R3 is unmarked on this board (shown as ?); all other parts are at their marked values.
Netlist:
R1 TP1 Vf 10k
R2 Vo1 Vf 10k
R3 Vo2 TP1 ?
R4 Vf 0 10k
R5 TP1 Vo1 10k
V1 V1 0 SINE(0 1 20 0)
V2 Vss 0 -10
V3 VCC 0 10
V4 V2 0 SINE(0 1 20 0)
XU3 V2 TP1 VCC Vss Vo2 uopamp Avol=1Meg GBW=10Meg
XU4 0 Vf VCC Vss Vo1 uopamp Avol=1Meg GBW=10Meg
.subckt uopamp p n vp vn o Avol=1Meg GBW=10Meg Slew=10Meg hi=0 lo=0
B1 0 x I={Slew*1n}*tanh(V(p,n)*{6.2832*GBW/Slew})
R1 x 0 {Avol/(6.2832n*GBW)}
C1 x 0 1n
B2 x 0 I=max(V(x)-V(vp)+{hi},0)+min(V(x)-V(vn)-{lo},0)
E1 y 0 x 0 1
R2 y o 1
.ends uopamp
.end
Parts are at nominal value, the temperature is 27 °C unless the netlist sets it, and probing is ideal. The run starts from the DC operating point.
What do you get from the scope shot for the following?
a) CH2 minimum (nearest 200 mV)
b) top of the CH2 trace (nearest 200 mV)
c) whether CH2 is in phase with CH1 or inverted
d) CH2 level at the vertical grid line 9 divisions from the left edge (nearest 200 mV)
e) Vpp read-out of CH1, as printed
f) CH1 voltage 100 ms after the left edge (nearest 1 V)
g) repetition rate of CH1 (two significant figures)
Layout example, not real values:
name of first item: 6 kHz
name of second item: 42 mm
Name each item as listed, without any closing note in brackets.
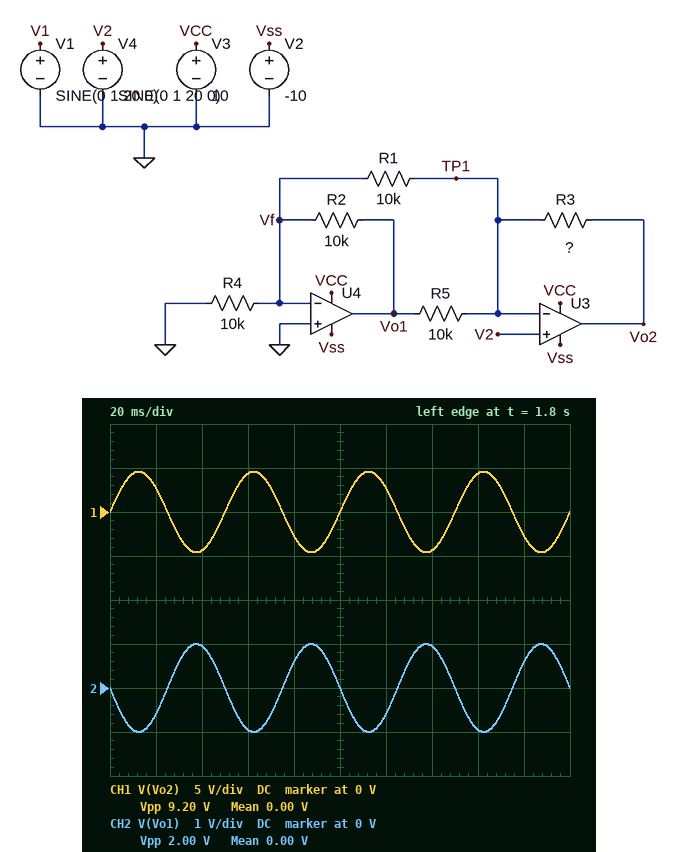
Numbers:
CH2 minimum: -1.0 V
top of the CH2 trace: 1.0 V
whether CH2 is in phase with CH1 or inverted: inverted
CH2 level at the vertical grid line 9 divisions from the left edge: 600 mV
Vpp read-out of CH1, as printed: 9.20 V
CH1 voltage 100 ms after the left edge: 0 V
repetition rate of CH1: 20 Hz
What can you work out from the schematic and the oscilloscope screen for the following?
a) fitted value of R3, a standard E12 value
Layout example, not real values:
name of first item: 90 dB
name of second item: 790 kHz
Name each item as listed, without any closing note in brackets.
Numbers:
fitted value of R3, a standard E12 value: 12 kΩ
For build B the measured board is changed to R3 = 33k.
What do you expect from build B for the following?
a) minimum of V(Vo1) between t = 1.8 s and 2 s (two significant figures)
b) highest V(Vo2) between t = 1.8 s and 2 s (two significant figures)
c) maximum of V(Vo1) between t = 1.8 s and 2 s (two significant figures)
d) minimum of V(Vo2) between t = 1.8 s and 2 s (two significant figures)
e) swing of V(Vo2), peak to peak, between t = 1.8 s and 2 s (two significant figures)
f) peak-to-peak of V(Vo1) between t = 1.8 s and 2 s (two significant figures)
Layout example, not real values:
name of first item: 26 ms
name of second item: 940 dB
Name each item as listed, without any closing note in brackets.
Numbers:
minimum of V(Vo1) between t = 1.8 s and 2 s: -920 mV
highest V(Vo2) between t = 1.8 s and 2 s: 10 V
maximum of V(Vo1) between t = 1.8 s and 2 s: 920 mV
minimum of V(Vo2) between t = 1.8 s and 2 s: -10 V
swing of V(Vo2), peak to peak, between t = 1.8 s and 2 s: 20 V
peak-to-peak of V(Vo1) between t = 1.8 s and 2 s: 1.8 V
